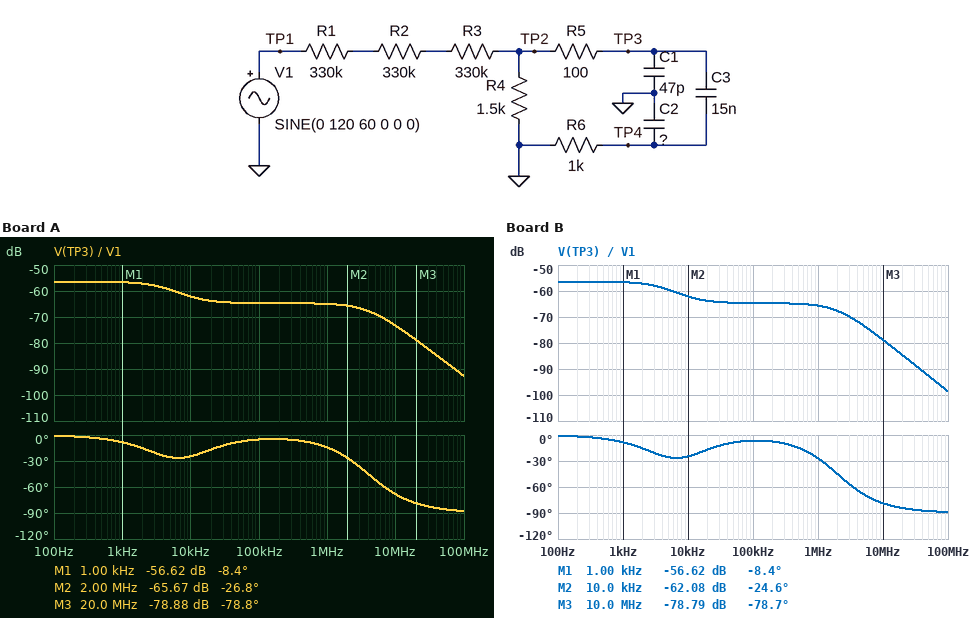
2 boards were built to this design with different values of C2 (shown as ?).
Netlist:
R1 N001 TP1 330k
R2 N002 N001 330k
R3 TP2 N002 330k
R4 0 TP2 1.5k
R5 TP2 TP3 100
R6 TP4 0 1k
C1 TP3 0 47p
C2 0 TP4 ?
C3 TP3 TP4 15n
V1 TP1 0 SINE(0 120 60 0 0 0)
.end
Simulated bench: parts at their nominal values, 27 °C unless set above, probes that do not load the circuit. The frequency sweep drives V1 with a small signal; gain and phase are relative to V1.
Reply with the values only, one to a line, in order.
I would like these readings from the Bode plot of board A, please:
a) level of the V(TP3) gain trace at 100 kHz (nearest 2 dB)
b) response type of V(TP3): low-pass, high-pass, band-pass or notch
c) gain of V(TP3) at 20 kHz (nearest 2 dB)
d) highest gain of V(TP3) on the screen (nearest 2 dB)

-64 dB
low-pass
-64 dB
-56 dB
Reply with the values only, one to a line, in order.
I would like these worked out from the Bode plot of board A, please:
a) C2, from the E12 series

18 pF
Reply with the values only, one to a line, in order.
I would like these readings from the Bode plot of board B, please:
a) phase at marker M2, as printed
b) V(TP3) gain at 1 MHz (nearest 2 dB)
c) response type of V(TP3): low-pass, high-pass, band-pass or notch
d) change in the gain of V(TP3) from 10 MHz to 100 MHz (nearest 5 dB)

-24.6 deg
-66 dB
low-pass
-20 dB
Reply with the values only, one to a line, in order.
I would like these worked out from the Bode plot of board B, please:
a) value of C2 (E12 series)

82 pF
